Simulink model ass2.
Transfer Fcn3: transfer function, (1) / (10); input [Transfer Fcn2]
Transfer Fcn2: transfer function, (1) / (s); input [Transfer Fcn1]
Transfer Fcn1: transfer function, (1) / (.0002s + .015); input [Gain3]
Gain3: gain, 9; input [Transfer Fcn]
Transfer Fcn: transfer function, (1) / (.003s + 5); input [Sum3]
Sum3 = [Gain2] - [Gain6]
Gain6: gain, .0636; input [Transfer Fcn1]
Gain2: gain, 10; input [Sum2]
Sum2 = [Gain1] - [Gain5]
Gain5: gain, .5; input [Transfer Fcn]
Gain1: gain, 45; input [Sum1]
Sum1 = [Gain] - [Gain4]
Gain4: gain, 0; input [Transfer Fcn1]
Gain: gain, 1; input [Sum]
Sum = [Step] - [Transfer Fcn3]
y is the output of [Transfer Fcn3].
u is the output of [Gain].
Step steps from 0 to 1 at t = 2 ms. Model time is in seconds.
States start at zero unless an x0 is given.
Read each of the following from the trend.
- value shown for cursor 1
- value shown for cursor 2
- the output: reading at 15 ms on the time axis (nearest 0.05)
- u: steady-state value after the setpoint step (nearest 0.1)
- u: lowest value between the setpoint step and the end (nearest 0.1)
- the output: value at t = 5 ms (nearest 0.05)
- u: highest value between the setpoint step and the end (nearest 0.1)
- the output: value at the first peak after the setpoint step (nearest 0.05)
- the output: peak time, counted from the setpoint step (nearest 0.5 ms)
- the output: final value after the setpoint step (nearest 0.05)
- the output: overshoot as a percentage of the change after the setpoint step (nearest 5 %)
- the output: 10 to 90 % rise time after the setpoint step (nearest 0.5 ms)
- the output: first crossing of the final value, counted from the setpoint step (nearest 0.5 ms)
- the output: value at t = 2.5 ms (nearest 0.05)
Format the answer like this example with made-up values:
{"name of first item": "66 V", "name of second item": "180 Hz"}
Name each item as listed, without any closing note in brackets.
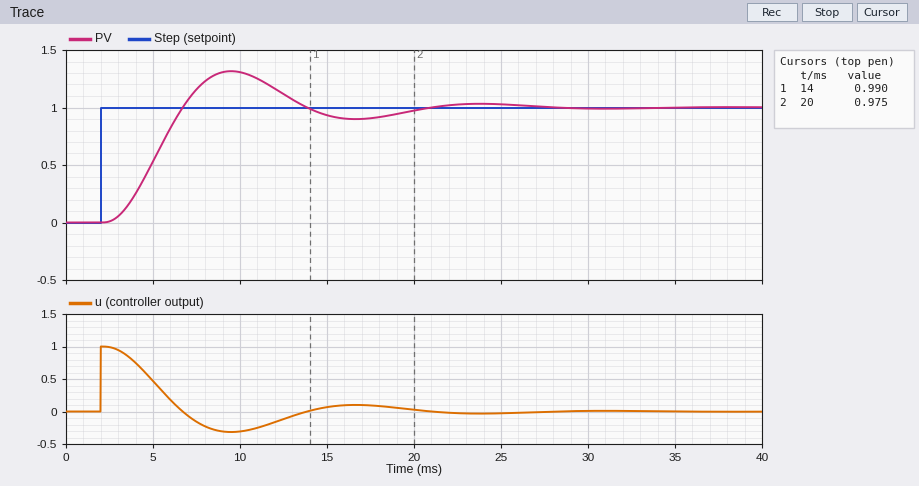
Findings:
{"value shown for cursor 1": "0.990", "value shown for cursor 2": "0.975", "the output: reading at 15 ms on the time axis": "0.95", "u: steady-state value after the setpoint step": "0.0", "u: lowest value between the setpoint step and the end": "-0.3", "the output: value at t = 5 ms": "0.55", "u: highest value between the setpoint step and the end": "1.0", "the output: value at the first peak after the setpoint step": "1.30", "the output: peak time, counted from the setpoint step": "7.5 ms", "the output: final value after the setpoint step": "1.00", "the output: overshoot as a percentage of the change after the setpoint step": "30 %", "the output: 10 to 90 % rise time after the setpoint step": "3.0 ms", "the output: first crossing of the final value, counted from the setpoint step": "4.5 ms", "the output: value at t = 2.5 ms": "0.00"}
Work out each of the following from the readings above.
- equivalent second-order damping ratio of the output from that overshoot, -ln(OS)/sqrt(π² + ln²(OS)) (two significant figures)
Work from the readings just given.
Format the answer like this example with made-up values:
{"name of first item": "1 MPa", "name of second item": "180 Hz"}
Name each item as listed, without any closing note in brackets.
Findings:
{"equivalent second-order damping ratio of the output from that overshoot, -ln(OS)/sqrt(π² + ln²(OS))": "0.36"}
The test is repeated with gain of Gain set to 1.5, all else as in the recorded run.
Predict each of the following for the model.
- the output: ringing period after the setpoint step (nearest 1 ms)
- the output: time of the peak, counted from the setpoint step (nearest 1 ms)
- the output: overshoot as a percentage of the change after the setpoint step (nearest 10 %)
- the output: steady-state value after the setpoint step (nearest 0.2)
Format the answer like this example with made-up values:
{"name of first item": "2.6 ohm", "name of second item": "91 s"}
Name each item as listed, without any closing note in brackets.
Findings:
{"the output: ringing period after the setpoint step": "11 ms", "the output: time of the peak, counted from the setpoint step": "6 ms", "the output: overshoot as a percentage of the change after the setpoint step": "40 %", "the output: steady-state value after the setpoint step": "1.0"}
